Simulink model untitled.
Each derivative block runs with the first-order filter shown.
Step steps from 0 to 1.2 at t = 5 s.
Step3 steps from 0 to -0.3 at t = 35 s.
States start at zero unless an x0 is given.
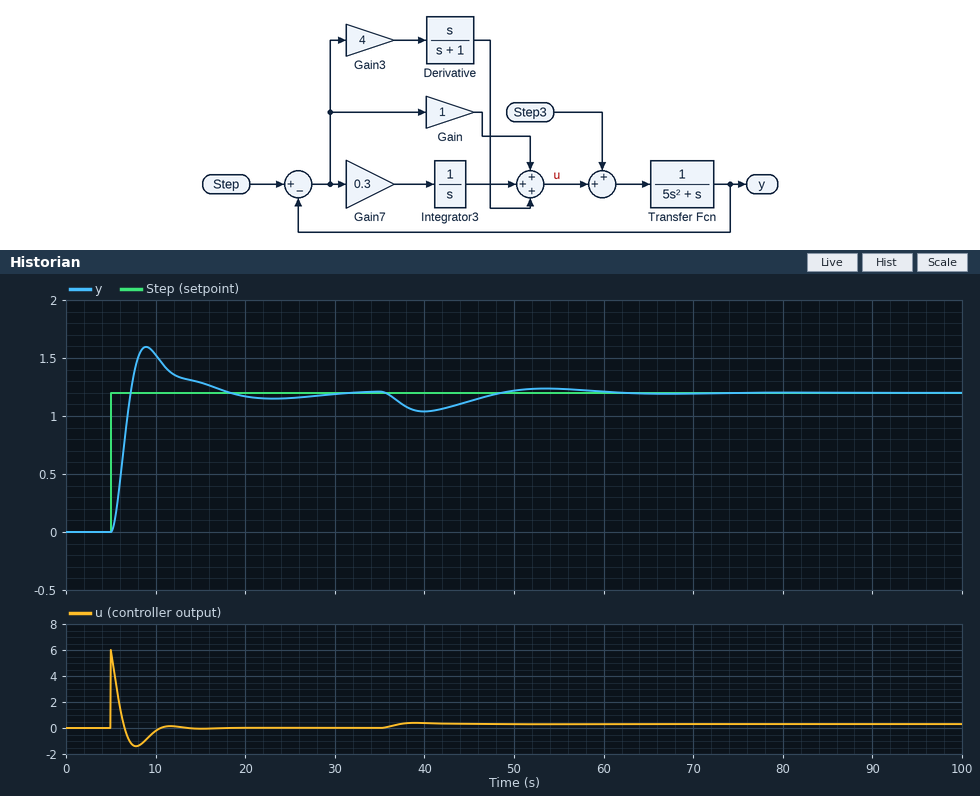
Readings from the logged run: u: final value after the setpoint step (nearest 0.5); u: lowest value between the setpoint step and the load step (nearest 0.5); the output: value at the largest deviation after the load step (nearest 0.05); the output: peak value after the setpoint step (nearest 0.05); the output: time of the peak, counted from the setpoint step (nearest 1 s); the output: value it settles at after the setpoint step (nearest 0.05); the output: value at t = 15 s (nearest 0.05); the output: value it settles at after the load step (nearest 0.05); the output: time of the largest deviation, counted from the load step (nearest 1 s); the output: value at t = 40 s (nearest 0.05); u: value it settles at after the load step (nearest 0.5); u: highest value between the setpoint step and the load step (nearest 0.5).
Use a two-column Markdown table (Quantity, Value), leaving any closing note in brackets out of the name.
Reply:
| Quantity | Value |
|---|---|
| u: final value after the setpoint step | 0.0 |
| u: lowest value between the setpoint step and the load step | -1.5 |
| the output: value at the largest deviation after the load step | 1.05 |
| the output: peak value after the setpoint step | 1.60 |
| the output: time of the peak, counted from the setpoint step | 4 s |
| the output: value it settles at after the setpoint step | 1.20 |
| the output: value at t = 15 s | 1.30 |
| the output: value it settles at after the load step | 1.20 |
| the output: time of the largest deviation, counted from the load step | 5 s |
| the output: value at t = 40 s | 1.05 |
| u: value it settles at after the load step | 0.5 |
| u: highest value between the setpoint step and the load step | 6.0 |
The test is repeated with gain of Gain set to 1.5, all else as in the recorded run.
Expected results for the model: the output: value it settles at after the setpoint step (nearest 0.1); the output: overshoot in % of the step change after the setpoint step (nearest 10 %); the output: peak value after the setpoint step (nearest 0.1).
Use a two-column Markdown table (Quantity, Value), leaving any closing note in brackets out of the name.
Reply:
| Quantity | Value |
|---|---|
| the output: value it settles at after the setpoint step | 1.2 |
| the output: overshoot in % of the step change after the setpoint step | 40 % |
| the output: peak value after the setpoint step | 1.7 |
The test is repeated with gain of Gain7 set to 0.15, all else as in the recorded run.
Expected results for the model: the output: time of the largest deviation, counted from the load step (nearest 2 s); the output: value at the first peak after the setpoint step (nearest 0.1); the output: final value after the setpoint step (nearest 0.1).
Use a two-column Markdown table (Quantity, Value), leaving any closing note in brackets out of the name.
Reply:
| Quantity | Value |
|---|---|
| the output: time of the largest deviation, counted from the load step | 6 s |
| the output: value at the first peak after the setpoint step | 1.5 |
| the output: final value after the setpoint step | 1.2 |
